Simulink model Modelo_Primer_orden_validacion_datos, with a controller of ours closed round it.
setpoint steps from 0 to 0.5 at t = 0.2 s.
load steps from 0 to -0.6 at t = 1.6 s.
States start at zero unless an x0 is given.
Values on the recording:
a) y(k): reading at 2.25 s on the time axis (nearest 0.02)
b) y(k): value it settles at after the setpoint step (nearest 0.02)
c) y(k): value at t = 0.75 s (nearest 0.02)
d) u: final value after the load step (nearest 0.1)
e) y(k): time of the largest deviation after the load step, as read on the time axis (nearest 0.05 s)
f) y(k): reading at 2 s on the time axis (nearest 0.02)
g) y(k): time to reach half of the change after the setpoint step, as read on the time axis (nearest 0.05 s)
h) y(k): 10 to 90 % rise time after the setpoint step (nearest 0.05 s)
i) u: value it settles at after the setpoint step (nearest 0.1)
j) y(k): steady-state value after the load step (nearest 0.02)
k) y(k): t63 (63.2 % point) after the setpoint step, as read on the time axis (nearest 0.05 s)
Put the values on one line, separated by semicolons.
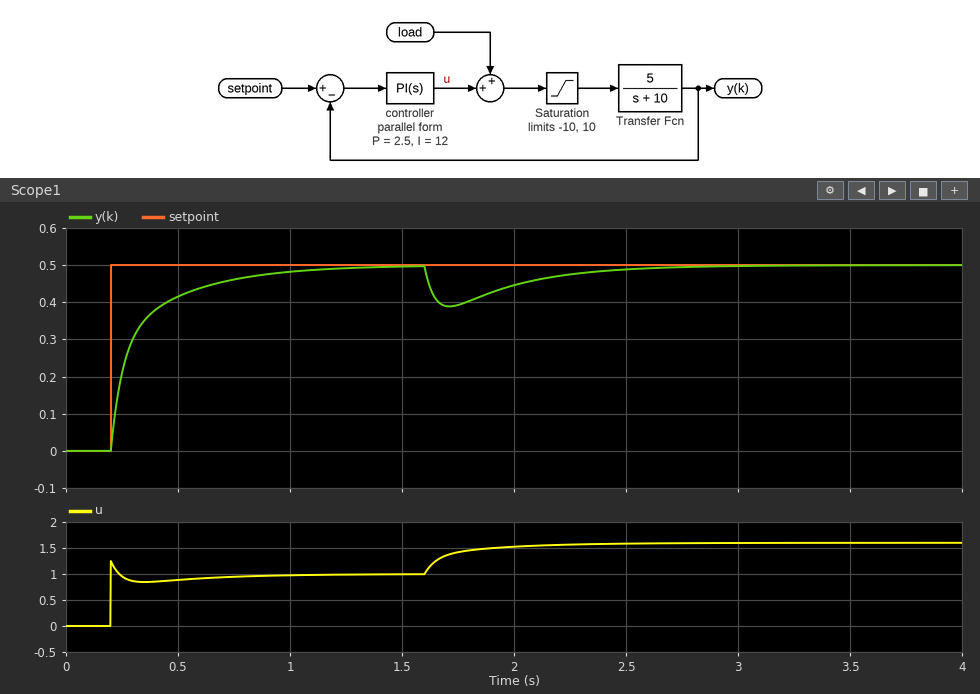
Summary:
0.48; 0.50; 0.46; 1.6; 1.70 s; 0.44; 0.25 s; 0.45 s; 1.0; 0.50; 0.30 s
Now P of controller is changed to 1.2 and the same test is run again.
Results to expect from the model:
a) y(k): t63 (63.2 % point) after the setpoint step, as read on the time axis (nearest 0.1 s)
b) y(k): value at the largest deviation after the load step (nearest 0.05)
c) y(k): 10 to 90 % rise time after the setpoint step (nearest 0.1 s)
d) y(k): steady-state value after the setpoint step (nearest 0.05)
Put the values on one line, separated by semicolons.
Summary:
0.4 s; 0.35; 0.4 s; 0.50
